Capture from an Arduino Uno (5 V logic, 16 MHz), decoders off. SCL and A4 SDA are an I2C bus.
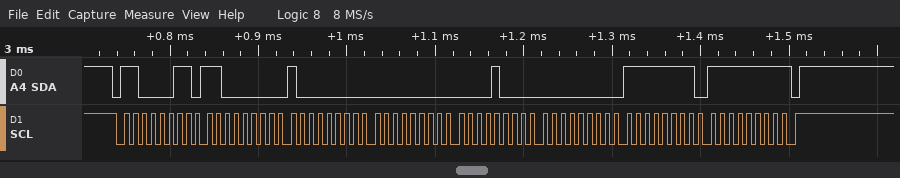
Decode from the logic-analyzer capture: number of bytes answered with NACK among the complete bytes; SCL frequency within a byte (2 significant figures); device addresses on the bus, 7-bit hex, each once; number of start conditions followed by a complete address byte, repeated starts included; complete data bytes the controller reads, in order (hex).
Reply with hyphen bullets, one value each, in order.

- 1
- 100 kHz
- 0x61
- 1
- C0 80 00 08 00 FF FF
